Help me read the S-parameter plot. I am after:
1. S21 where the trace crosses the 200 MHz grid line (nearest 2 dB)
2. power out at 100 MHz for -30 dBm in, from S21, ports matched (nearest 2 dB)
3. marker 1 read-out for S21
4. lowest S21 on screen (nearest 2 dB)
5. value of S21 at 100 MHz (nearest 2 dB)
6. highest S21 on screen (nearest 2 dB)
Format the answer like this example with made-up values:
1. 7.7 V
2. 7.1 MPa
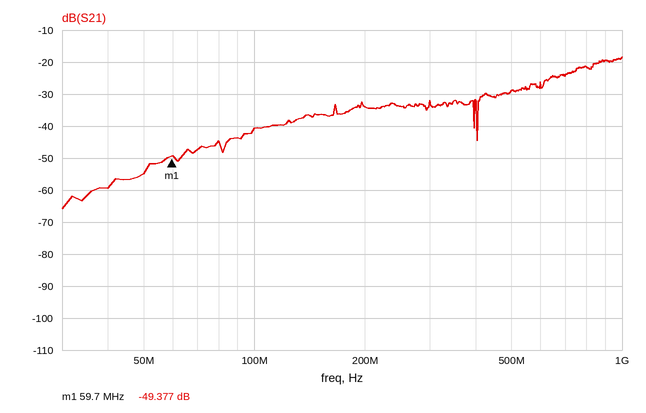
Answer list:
1. -34 dB
2. -70 dBm
3. -49.377 dB
4. -66 dB
5. -40 dB
6. -18 dB
